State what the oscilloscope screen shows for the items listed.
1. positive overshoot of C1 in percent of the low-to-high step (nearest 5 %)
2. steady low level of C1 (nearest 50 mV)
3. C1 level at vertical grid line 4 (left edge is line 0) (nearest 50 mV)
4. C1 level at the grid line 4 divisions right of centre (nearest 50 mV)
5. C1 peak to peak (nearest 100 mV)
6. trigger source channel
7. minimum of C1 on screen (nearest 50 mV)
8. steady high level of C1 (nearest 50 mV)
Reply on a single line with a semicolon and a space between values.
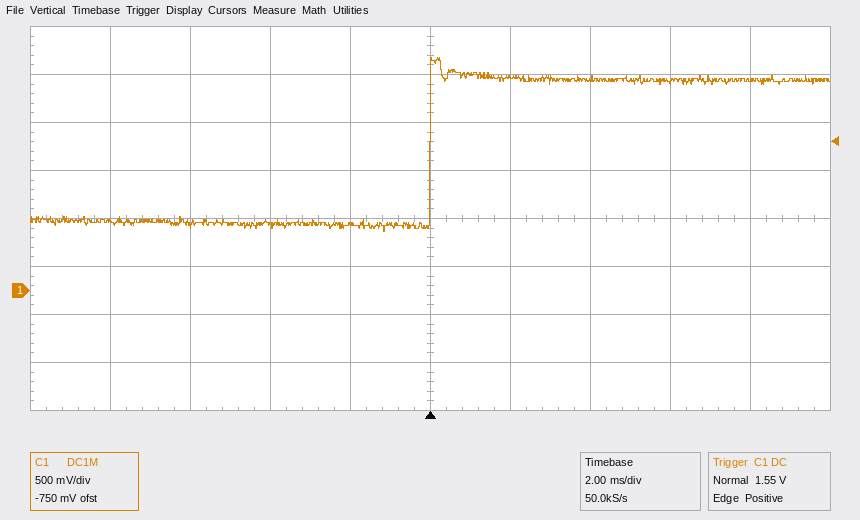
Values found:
15 %; 700 mV; 700 mV; 2.20 V; 1.80 V; C1; 600 mV; 2.20 V
